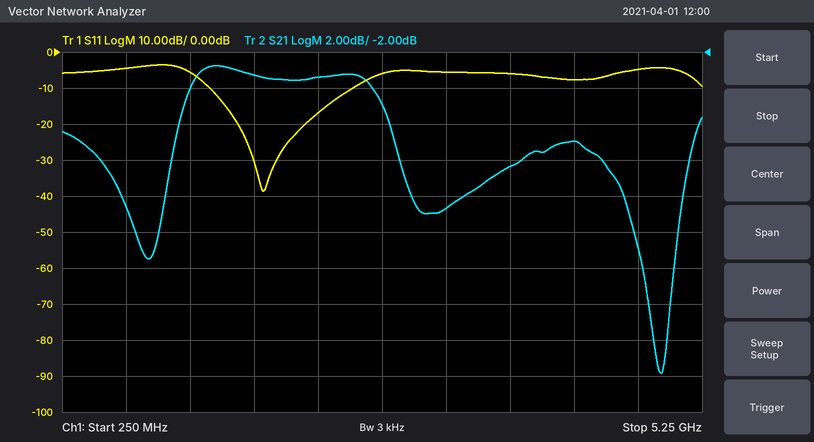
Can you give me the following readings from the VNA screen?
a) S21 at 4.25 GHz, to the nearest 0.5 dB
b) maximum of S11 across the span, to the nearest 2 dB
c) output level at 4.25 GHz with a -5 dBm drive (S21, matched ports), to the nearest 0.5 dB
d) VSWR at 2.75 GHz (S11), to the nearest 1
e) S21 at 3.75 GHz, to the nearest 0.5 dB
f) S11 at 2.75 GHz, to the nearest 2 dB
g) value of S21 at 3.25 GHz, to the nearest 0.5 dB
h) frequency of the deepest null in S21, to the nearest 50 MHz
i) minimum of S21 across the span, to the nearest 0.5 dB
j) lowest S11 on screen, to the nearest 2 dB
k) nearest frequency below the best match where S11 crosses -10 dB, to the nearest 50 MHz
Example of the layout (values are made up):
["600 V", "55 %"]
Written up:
["-7.0 dB", "-4 dB", "-12.0 dBm", "3", "-8.5 dB", "-6 dB", "-10.5 dB", "4.95 GHz", "-20.0 dB", "-38 dB", "1.40 GHz"]
